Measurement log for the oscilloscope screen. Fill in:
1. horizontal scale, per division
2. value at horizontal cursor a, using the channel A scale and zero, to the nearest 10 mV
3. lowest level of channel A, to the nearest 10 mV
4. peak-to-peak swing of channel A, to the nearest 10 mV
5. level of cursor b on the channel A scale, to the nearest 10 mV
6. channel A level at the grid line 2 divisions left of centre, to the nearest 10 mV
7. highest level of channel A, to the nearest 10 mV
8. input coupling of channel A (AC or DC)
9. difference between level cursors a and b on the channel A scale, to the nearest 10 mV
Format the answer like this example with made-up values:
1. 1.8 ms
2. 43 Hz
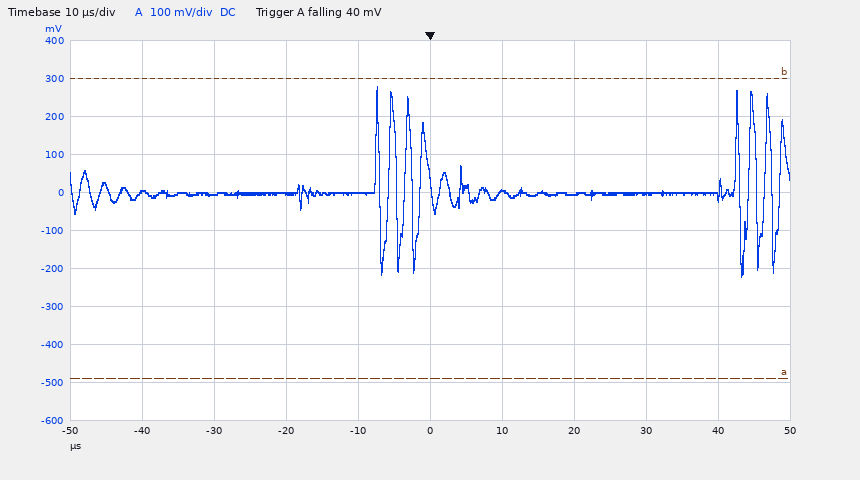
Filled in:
1. 10 µs
2. -490 mV
3. -220 mV
4. 500 mV
5. 300 mV
6. 0 mV
7. 280 mV
8. DC
9. 790 mV
